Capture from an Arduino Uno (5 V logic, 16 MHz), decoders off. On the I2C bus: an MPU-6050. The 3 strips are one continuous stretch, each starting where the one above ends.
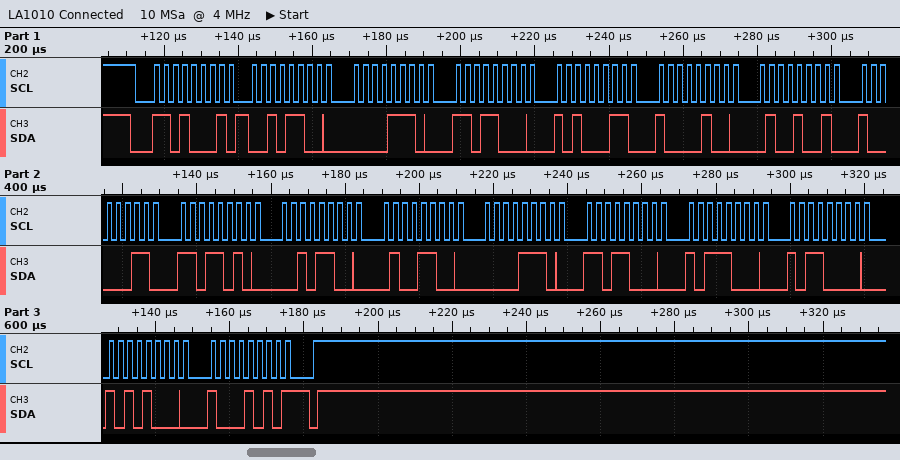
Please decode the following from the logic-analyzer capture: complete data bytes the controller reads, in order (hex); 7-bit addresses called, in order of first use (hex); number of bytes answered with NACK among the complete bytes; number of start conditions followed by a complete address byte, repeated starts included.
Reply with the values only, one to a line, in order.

2C 0E D8 A3 84 49 83 DA 2C 4C 0E D8 B8 B0 A8 8A
0x68
1
1
